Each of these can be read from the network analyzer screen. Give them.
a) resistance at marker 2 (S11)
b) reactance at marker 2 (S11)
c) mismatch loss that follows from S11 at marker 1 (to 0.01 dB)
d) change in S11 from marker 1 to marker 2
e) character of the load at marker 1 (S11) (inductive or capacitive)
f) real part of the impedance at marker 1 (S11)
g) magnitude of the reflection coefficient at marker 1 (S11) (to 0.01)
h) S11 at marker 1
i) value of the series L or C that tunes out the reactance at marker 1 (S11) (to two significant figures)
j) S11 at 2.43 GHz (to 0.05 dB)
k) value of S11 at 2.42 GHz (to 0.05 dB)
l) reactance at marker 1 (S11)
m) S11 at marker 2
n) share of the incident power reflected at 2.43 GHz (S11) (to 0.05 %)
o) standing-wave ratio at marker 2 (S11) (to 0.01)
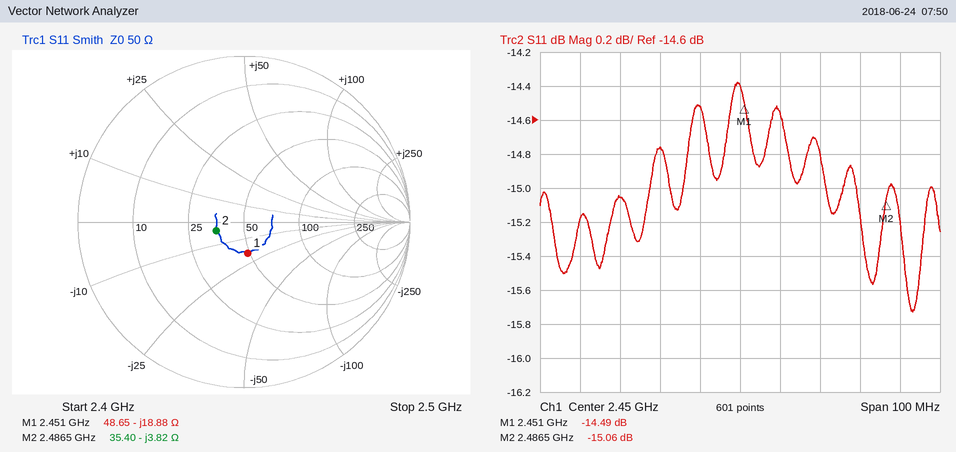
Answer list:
35.40 Ω
-3.82 Ω
0.16 dB
-0.57 dB
capacitive
48.65 Ω
0.19
-14.49 dB
1.2 nH
-14.75 dB
-15.05 dB
-18.88 Ω
-15.06 dB
3.35 %
1.43
